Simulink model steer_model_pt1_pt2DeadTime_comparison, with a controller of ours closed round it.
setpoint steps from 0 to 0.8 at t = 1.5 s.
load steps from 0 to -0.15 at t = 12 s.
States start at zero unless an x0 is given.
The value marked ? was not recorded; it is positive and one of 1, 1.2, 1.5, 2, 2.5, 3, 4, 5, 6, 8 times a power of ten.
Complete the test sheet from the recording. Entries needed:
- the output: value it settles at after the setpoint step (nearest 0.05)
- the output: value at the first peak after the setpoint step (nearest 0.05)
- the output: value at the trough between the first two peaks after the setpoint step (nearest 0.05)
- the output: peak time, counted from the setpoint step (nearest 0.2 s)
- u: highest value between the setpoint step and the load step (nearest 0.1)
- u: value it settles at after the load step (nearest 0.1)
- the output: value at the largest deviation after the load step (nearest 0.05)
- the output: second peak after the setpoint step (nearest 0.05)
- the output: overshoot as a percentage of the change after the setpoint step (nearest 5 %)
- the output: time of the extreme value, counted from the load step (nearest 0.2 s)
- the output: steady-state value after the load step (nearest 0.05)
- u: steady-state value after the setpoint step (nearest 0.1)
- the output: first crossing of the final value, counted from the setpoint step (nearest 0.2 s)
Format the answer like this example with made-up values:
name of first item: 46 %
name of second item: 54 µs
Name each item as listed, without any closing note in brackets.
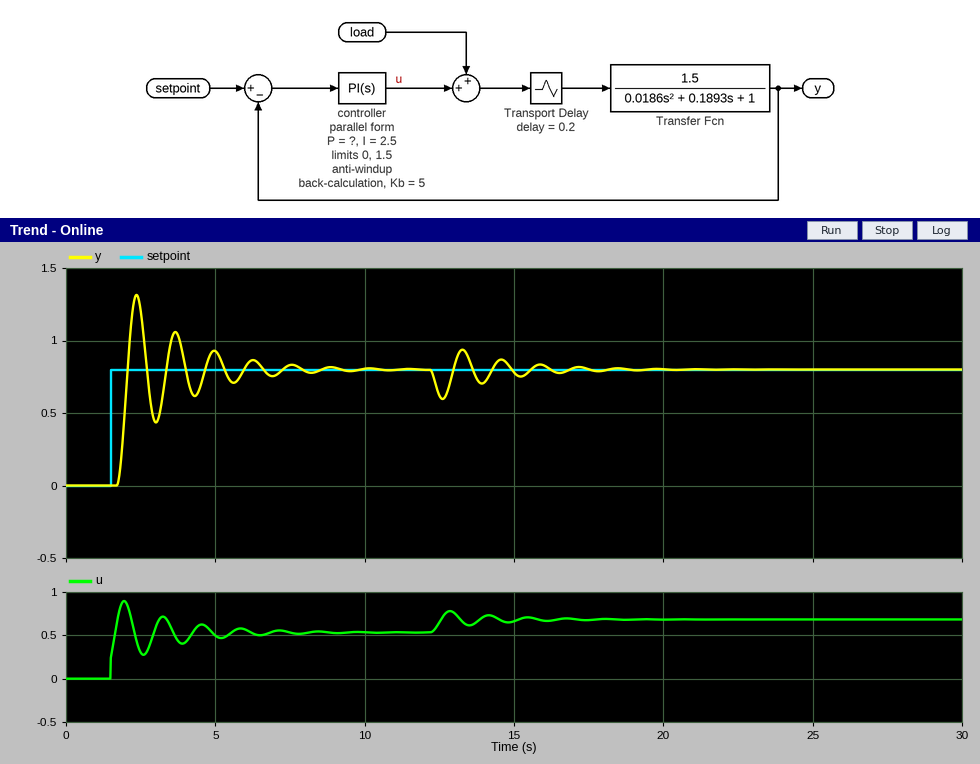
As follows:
the output: value it settles at after the setpoint step: 0.80
the output: value at the first peak after the setpoint step: 1.30
the output: value at the trough between the first two peaks after the setpoint step: 0.45
the output: peak time, counted from the setpoint step: 0.8 s
u: highest value between the setpoint step and the load step: 0.9
u: value it settles at after the load step: 0.7
the output: value at the largest deviation after the load step: 0.60
the output: second peak after the setpoint step: 1.05
the output: overshoot as a percentage of the change after the setpoint step: 65 %
the output: time of the extreme value, counted from the load step: 0.6 s
the output: steady-state value after the load step: 0.80
u: steady-state value after the setpoint step: 0.5
the output: first crossing of the final value, counted from the setpoint step: 0.6 s
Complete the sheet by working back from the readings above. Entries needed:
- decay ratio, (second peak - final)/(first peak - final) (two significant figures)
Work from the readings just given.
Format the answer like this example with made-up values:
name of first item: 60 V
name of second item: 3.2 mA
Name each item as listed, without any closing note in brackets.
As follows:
decay ratio, (second peak - final)/(first peak - final): 0.50
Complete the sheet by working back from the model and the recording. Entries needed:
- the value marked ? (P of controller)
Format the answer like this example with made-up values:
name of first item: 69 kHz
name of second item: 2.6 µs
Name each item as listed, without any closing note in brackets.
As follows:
the value marked ?: 0.3
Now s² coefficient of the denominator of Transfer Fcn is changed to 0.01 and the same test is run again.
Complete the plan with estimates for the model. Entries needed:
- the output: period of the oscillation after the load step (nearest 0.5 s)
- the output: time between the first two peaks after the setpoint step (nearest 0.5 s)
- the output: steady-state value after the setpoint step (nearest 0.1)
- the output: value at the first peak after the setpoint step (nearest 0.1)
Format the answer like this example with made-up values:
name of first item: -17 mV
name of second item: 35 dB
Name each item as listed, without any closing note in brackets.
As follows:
the output: period of the oscillation after the load step: 1.5 s
the output: time between the first two peaks after the setpoint step: 1.5 s
the output: steady-state value after the setpoint step: 0.8
the output: value at the first peak after the setpoint step: 1.2
